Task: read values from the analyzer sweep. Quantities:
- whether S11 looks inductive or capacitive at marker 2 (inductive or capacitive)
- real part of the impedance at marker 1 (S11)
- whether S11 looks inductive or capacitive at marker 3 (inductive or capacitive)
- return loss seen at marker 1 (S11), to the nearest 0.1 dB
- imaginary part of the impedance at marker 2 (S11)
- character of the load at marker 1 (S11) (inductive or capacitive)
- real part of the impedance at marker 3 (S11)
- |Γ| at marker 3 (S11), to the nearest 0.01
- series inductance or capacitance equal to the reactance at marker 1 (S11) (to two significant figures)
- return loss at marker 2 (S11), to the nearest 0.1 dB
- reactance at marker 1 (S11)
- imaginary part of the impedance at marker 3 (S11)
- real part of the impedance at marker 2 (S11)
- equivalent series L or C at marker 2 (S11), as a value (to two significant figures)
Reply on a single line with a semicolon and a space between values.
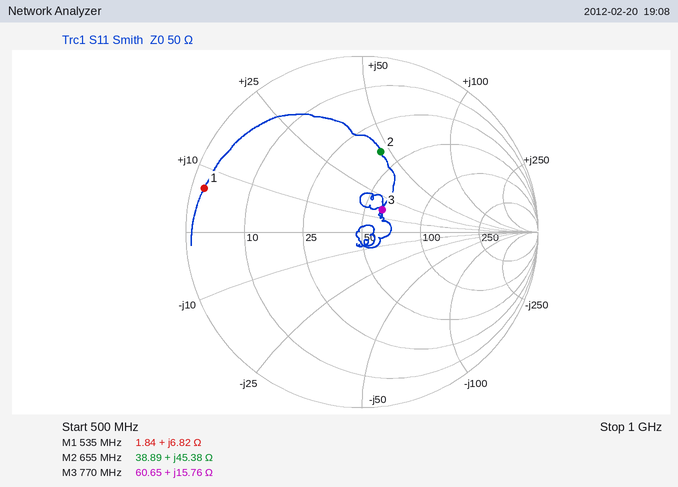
inductive; 1.84 Ω; inductive; 0.6 dB; +45.38 Ω; inductive; 60.65 Ω; 0.17; 2.0 nH; 6.6 dB; +6.82 Ω; +15.76 Ω; 38.89 Ω; 11 nH
